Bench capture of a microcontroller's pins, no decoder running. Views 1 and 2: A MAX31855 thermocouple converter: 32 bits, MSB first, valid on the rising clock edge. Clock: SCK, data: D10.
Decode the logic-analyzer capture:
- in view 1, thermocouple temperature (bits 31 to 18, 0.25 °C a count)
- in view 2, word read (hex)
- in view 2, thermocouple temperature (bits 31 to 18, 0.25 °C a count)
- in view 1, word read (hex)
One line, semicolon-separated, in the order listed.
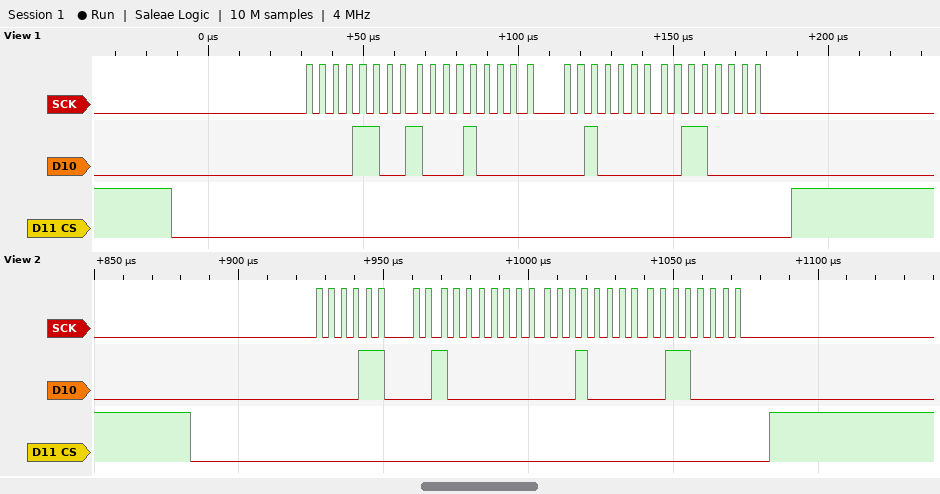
200.50 °C; 0x0C801030; 200.00 °C; 0x0C881030
